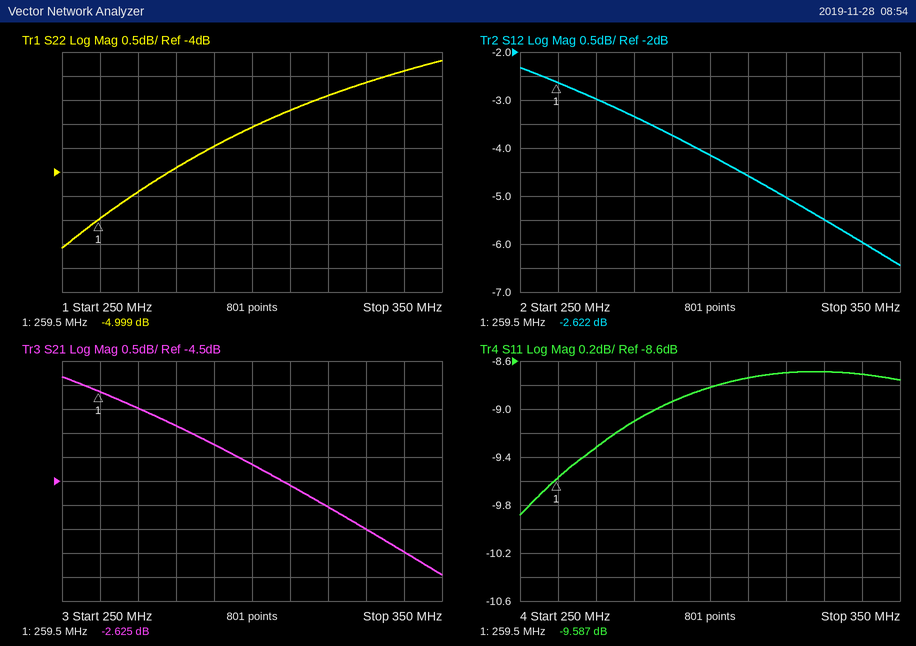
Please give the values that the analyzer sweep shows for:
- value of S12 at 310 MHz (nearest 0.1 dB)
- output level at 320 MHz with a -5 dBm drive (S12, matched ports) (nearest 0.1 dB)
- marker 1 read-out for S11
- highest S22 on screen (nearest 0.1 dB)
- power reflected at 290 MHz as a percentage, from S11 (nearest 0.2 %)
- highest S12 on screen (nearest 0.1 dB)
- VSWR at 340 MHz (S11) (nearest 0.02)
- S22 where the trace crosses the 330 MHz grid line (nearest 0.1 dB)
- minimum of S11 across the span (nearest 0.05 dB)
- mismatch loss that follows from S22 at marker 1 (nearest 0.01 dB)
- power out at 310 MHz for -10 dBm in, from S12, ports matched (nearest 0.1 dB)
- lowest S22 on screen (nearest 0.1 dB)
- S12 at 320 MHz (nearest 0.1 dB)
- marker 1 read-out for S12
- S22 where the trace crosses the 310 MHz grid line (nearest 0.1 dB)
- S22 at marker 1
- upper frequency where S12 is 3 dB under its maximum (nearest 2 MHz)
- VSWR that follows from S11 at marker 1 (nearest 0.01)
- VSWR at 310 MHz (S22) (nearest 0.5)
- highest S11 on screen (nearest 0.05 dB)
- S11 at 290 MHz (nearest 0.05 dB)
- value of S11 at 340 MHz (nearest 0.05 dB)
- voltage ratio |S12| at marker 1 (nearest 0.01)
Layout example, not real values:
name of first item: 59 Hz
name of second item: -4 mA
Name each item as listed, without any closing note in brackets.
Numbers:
value of S12 at 310 MHz: -4.6 dB
output level at 320 MHz with a -5 dBm drive (S12, matched ports): -10.0 dBm
marker 1 read-out for S11: -9.587 dB
highest S22 on screen: -1.7 dB
power reflected at 290 MHz as a percentage, from S11: 12.8 %
highest S12 on screen: -2.3 dB
VSWR at 340 MHz (S11): 2.16
S22 where the trace crosses the 330 MHz grid line: -2.1 dB
minimum of S11 across the span: -9.90 dB
mismatch loss that follows from S22 at marker 1: 1.65 dB
power out at 310 MHz for -10 dBm in, from S12, ports matched: -14.6 dBm
lowest S22 on screen: -5.6 dB
S12 at 320 MHz: -5.0 dB
marker 1 read-out for S12: -2.622 dB
S22 where the trace crosses the 310 MHz grid line: -2.7 dB
S22 at marker 1: -4.999 dB
upper frequency where S12 is 3 dB under its maximum: 326 MHz
VSWR that follows from S11 at marker 1: 1.99
VSWR at 310 MHz (S22): 6.5
highest S11 on screen: -8.70 dB
S11 at 290 MHz: -8.95 dB
value of S11 at 340 MHz: -8.70 dB
voltage ratio |S12| at marker 1: 0.74
